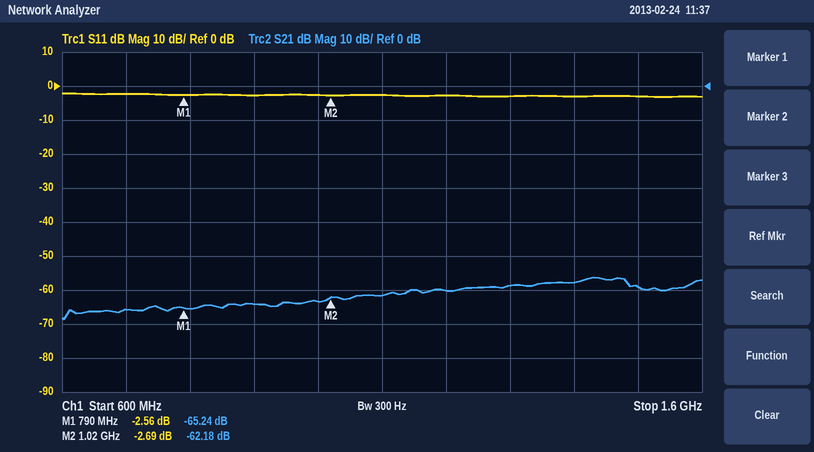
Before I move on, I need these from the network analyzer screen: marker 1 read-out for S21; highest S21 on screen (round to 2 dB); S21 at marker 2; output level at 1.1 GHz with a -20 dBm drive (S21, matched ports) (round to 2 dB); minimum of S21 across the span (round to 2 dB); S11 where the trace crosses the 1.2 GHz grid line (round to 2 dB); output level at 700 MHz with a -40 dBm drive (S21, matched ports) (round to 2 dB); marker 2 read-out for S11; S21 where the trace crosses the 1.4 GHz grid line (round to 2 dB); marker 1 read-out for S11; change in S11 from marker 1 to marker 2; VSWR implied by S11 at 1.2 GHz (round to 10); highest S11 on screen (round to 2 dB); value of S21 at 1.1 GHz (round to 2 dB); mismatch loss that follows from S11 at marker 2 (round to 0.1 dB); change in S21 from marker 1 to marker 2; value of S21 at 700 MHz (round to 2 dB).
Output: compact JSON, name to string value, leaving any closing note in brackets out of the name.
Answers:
{"marker 1 read-out for S21": "-65.24 dB", "highest S21 on screen": "-56 dB", "S21 at marker 2": "-62.18 dB", "output level at 1.1 GHz with a -20 dBm drive (S21, matched ports)": "-82 dBm", "minimum of S21 across the span": "-68 dB", "S11 where the trace crosses the 1.2 GHz grid line": "-2 dB", "output level at 700 MHz with a -40 dBm drive (S21, matched ports)": "-106 dBm", "marker 2 read-out for S11": "-2.69 dB", "S21 where the trace crosses the 1.4 GHz grid line": "-58 dB", "marker 1 read-out for S11": "-2.56 dB", "change in S11 from marker 1 to marker 2": "-0.13 dB", "VSWR implied by S11 at 1.2 GHz": "10", "highest S11 on screen": "-2 dB", "value of S21 at 1.1 GHz": "-62 dB", "mismatch loss that follows from S11 at marker 2": "3.4 dB", "change in S21 from marker 1 to marker 2": "3.06 dB", "value of S21 at 700 MHz": "-66 dB"}
